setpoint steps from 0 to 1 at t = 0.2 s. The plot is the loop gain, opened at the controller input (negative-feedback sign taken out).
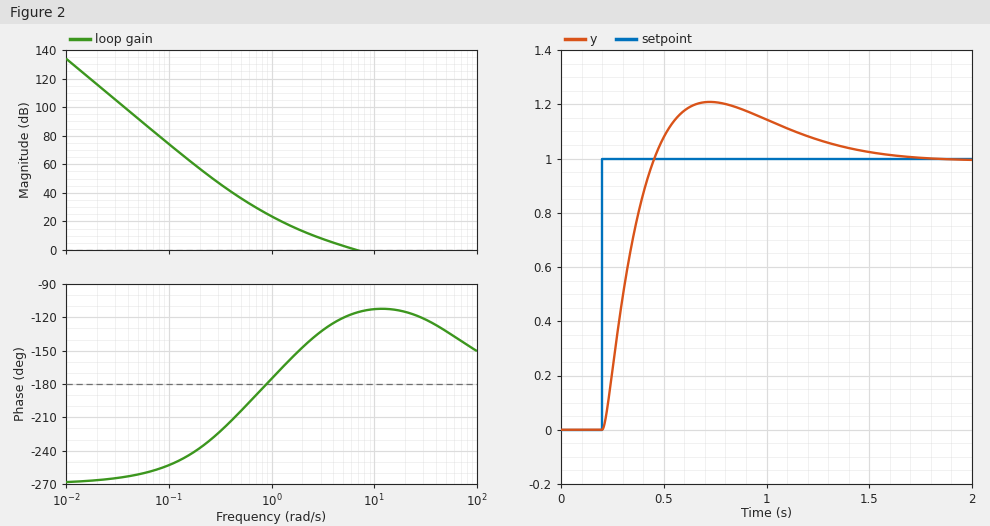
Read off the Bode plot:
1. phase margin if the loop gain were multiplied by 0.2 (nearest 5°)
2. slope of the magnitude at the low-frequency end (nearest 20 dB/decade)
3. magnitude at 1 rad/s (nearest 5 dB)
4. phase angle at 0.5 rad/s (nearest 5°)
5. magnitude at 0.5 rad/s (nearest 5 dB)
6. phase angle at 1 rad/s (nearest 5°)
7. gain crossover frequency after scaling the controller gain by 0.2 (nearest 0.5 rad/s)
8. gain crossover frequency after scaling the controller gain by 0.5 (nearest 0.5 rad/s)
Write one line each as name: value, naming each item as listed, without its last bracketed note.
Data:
phase margin if the loop gain were multiplied by 0.2: 30°
slope of the magnitude at the low-frequency end: -60 dB/decade
magnitude at 1 rad/s: 25 dB
phase angle at 0.5 rad/s: -205°
magnitude at 0.5 rad/s: 35 dB
phase angle at 1 rad/s: -175°
gain crossover frequency after scaling the controller gain by 0.2: 2.0 rad/s
gain crossover frequency after scaling the controller gain by 0.5: 3.5 rad/s
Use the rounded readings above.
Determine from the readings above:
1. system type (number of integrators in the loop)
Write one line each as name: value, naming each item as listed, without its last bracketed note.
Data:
system type: 3
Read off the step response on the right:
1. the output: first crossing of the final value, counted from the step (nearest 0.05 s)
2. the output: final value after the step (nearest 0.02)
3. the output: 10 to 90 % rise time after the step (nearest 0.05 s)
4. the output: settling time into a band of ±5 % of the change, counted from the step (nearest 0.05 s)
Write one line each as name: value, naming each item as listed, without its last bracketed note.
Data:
the output: first crossing of the final value, counted from the step: 0.25 s
the output: final value after the step: 1.00
the output: 10 to 90 % rise time after the step: 0.20 s
the output: settling time into a band of ±5 % of the change, counted from the step: 1.15 s
